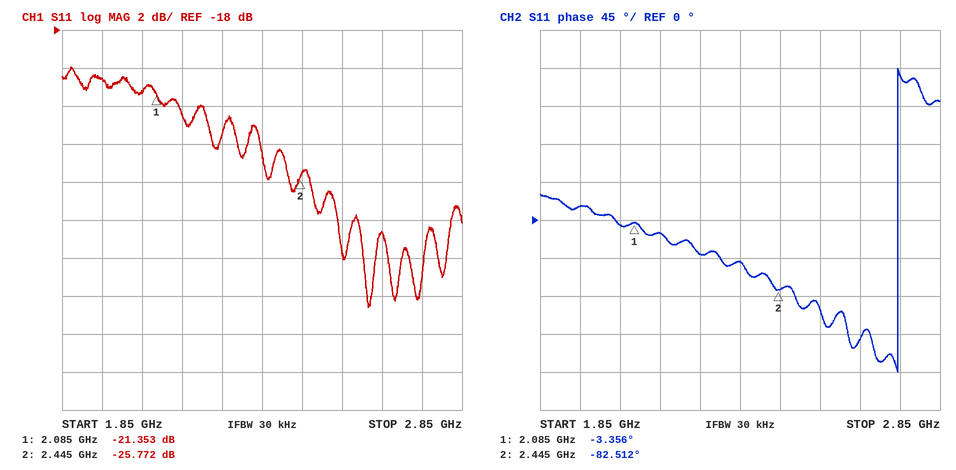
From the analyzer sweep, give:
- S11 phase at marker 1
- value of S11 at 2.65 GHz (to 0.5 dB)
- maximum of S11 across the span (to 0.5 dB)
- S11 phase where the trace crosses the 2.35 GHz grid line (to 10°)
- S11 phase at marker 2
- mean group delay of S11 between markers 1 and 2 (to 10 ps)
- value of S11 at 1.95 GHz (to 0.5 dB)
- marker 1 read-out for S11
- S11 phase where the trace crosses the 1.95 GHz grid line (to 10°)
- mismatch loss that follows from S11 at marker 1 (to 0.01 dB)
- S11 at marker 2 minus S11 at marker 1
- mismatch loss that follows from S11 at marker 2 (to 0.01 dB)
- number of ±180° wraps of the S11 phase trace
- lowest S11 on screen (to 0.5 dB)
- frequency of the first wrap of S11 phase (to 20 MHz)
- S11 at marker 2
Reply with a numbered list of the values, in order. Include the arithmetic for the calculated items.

1. -3.356°
2. -28.5 dB
3. -20.0 dB
4. -50°
5. -82.512°
6. −(-82.512° − (-3.356°))/(360° × 360 MHz) ≈ 611 ps, so 610 ps to the nearest 10 ps
7. -20.5 dB
8. -21.353 dB
9. 20°
10. −10 log10(1 − 10^(-21.353/10)) ≈ 0.03 dB
11. -25.772 − (-21.353) = -4.419 dB
12. −10 log10(1 − 10^(-25.772/10)) ≈ 0.01 dB
13. 1
14. -32.5 dB
15. 2.74 GHz
16. -25.772 dB
